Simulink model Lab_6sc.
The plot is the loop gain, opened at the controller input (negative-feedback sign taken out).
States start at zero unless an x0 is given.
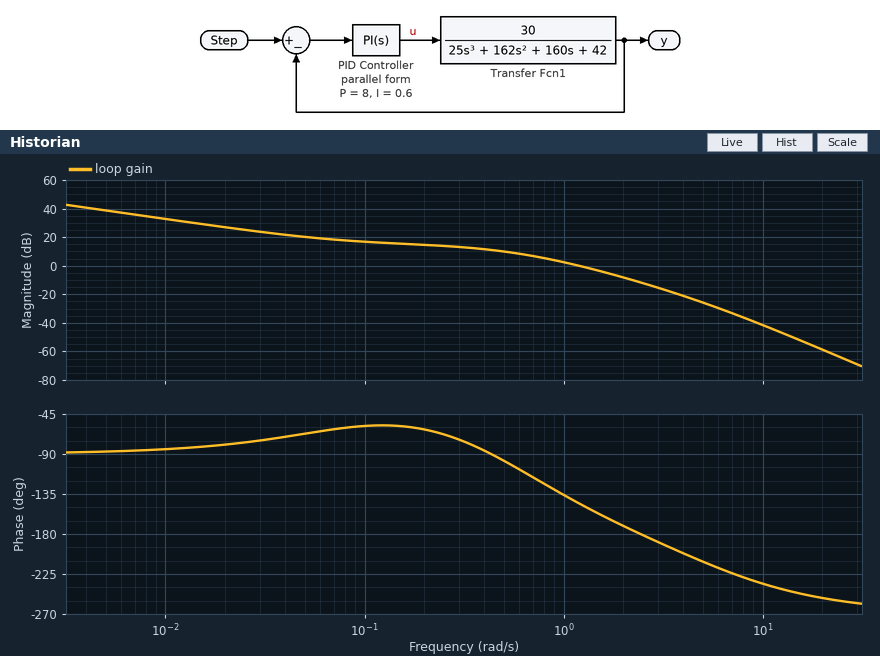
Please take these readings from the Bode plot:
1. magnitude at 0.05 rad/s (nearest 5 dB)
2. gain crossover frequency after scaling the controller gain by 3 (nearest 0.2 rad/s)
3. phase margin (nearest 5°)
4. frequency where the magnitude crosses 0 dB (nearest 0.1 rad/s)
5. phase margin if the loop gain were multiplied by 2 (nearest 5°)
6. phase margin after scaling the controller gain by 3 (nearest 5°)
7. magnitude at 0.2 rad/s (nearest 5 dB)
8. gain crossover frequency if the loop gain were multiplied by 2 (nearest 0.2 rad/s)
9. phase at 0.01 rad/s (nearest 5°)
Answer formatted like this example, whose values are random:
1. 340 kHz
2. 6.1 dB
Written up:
1. 20 dB
2. 2.2 rad/s
3. 35°
4. 1.2 rad/s
5. 15°
6. 5°
7. 15 dB
8. 1.8 rad/s
9. -85°
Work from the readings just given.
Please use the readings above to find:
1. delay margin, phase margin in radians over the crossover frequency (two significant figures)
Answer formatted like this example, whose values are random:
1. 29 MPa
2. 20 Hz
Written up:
1. 0.51 s
